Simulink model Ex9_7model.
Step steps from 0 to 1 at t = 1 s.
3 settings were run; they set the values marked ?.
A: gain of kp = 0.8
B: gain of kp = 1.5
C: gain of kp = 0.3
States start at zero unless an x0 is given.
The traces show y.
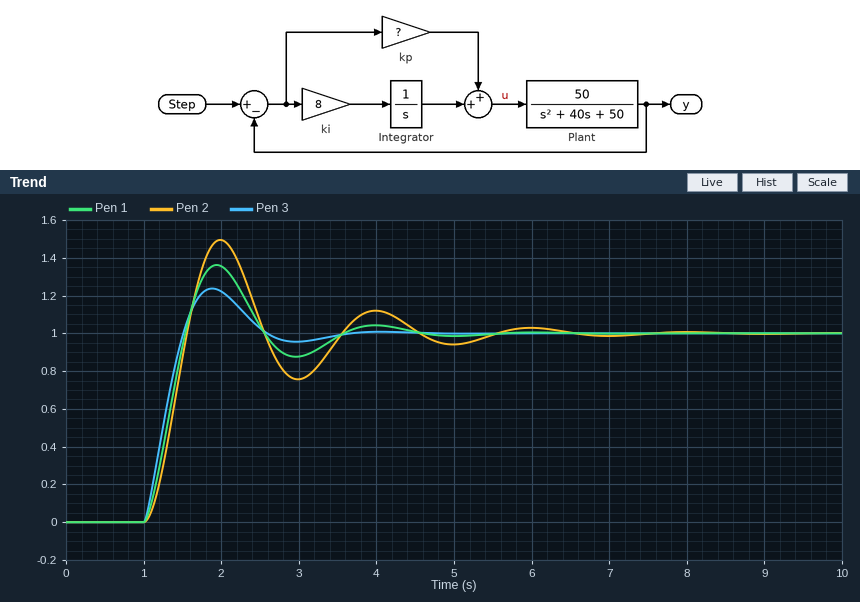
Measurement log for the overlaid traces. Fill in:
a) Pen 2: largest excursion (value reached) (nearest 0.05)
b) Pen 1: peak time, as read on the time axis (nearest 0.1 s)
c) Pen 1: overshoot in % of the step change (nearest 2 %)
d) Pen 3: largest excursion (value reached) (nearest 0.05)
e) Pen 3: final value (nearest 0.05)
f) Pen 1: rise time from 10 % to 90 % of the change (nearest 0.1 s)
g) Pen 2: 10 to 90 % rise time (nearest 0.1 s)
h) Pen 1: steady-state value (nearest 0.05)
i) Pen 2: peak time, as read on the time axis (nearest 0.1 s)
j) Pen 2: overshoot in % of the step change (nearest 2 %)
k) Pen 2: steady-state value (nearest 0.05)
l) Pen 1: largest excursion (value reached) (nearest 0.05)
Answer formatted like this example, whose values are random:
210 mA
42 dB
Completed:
1.50
1.9 s
36 %
1.25
1.00
0.4 s
0.4 s
1.00
2.0 s
50 %
1.00
1.35
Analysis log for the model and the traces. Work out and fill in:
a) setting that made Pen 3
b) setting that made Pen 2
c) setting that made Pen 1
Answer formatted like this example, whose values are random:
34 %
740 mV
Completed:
B
C
A
